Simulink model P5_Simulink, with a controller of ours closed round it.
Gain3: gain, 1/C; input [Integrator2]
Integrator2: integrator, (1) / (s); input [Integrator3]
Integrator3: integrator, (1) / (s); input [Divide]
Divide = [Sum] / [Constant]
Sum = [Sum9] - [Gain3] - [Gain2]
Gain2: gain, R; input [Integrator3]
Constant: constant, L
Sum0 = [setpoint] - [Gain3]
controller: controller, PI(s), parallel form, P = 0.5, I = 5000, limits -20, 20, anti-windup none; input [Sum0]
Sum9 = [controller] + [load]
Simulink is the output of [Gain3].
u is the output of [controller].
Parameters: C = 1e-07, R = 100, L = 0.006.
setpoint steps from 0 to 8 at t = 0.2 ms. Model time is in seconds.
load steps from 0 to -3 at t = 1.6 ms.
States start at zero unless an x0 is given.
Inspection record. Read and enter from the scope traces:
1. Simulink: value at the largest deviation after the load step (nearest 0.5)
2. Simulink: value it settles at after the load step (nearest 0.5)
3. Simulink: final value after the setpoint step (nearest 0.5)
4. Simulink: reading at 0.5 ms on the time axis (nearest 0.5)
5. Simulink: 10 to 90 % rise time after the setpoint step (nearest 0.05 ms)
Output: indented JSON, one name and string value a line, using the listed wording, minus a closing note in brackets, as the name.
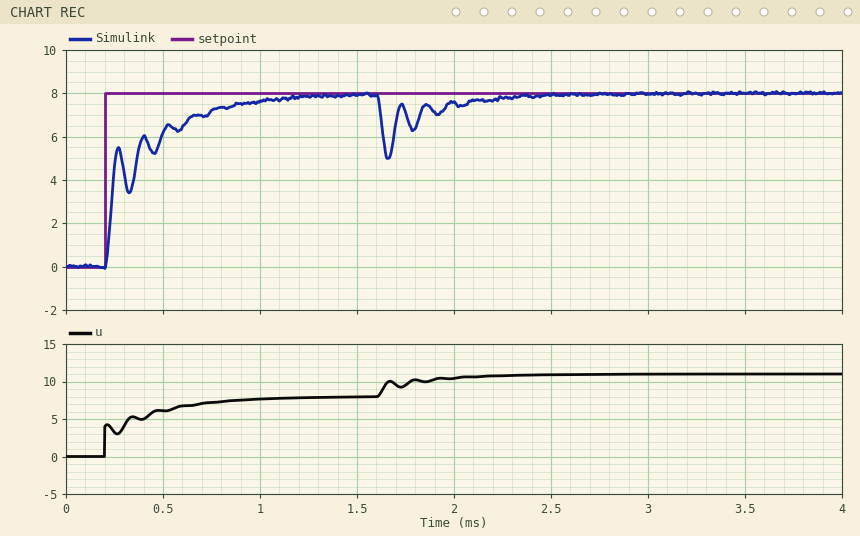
{
  "Simulink: value at the largest deviation after the load step": "5.0",
  "Simulink: value it settles at after the load step": "8.0",
  "Simulink: final value after the setpoint step": "8.0",
  "Simulink: reading at 0.5 ms on the time axis": "6.0",
  "Simulink: 10 to 90 % rise time after the setpoint step": "0.55 ms"
}
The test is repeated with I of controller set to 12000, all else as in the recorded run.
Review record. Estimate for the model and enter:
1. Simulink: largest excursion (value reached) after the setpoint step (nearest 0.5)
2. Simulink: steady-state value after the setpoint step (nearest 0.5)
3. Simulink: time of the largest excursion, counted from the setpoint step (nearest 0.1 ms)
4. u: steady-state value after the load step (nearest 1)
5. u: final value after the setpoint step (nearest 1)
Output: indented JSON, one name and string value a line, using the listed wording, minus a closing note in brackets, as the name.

{
  "Simulink: largest excursion (value reached) after the setpoint step": "8.5",
  "Simulink: steady-state value after the setpoint step": "8.0",
  "Simulink: time of the largest excursion, counted from the setpoint step": "0.3 ms",
  "u: steady-state value after the load step": "11",
  "u: final value after the setpoint step": "8"
}
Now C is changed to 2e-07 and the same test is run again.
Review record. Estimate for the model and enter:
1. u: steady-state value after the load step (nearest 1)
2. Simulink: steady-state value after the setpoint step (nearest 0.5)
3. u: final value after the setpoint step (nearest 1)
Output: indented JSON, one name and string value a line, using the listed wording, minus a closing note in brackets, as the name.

{
  "u: steady-state value after the load step": "11",
  "Simulink: steady-state value after the setpoint step": "8.0",
  "u: final value after the setpoint step": "8"
}
